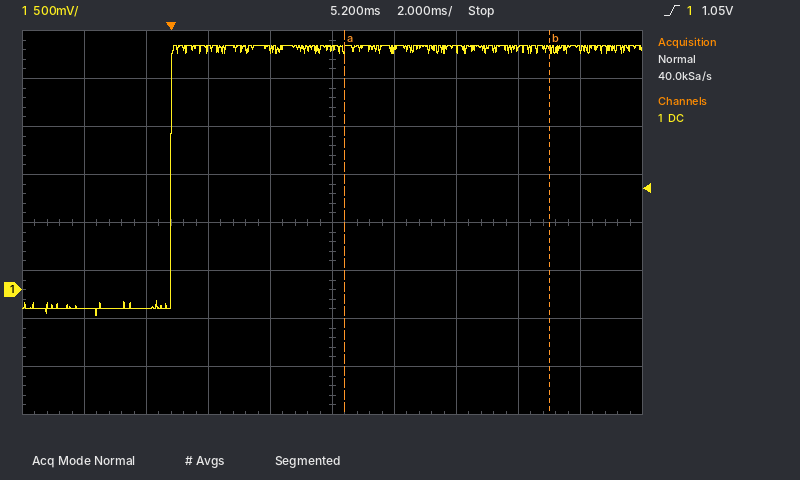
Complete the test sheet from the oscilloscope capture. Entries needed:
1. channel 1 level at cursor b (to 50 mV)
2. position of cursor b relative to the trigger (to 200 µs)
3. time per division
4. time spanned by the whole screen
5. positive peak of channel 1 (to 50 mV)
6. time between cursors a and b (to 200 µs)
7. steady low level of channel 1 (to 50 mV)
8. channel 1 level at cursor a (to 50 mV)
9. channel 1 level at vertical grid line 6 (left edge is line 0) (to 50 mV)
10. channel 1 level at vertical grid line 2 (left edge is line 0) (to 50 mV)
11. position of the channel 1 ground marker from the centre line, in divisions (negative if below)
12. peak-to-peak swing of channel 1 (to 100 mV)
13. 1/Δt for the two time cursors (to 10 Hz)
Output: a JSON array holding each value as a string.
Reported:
["2.50 V", "+12.2 ms", "2 ms", "20 ms", "2.55 V", "6.6 ms", "-200 mV", "2.50 V", "2.50 V", "-200 mV", "-1.4 div", "2.80 V", "150 Hz"]
